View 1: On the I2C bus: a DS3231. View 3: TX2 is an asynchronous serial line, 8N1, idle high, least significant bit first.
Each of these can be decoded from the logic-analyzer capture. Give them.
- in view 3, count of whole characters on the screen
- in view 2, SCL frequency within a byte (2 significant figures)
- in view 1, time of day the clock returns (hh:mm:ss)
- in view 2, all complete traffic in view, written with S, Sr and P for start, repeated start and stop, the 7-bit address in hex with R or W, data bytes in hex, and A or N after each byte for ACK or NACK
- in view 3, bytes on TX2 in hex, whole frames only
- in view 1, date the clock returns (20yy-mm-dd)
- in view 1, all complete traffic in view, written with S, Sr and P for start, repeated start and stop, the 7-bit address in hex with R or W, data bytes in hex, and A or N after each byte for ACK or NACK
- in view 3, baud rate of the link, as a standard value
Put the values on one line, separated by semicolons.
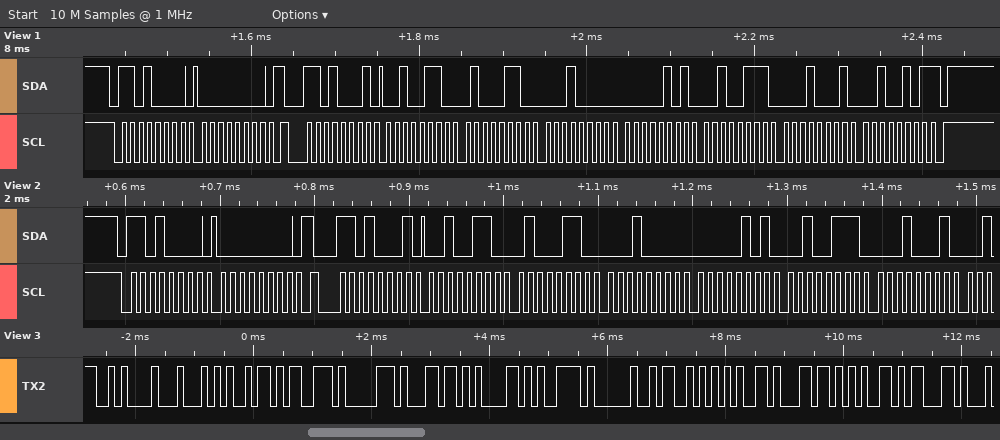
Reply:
14; 100 kHz; 10:46:26; S 68W A 00 A Sr 68R A 26 A 46 A 10 A 05 A 27 A 11 A; 0A 44 69 73 70 6C 61 79 20 53 65 6C 65 63; 2025-11-27; S 68W A 00 A Sr 68R A 26 A 46 A 10 A 05 A 27 A 11 A 25 N P; 9600 baud
